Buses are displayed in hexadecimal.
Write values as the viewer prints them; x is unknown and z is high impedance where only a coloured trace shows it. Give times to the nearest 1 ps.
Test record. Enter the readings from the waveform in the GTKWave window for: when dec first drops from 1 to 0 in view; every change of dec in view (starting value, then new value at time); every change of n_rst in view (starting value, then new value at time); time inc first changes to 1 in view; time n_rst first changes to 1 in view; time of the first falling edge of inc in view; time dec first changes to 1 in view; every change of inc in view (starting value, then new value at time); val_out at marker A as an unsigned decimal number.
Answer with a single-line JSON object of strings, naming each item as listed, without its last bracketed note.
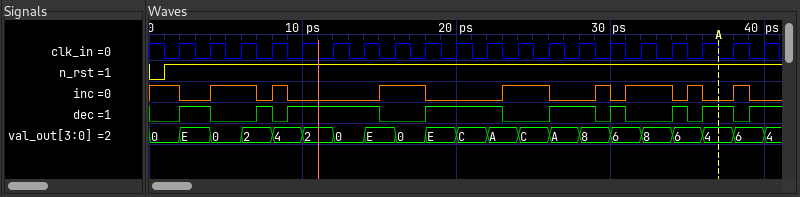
{"when dec first drops from 1 to 0 in view": "4 ps", "every change of dec in view": "0, 1 at 2 ps, 0 at 4 ps, 1 at 7 ps, 0 at 8 ps, 1 at 9 ps, 0 at 15 ps, 1 at 18 ps, 0 at 23 ps, 1 at 26 ps, 0 at 29 ps, 1 at 30 ps, 0 at 31 ps, 1 at 34 ps, 0 at 35 ps, 1 at 36 ps, 0 at 38 ps, 1 at 39 ps", "every change of n_rst in view": "0, 1 at 1 ps", "time inc first changes to 1 in view": "4 ps", "time n_rst first changes to 1 in view": "1 ps", "time of the first falling edge of inc in view": "2 ps", "time dec first changes to 1 in view": "2 ps", "every change of inc in view": "1, 0 at 2 ps, 1 at 4 ps, 0 at 7 ps, 1 at 8 ps, 0 at 9 ps, 1 at 15 ps, 0 at 18 ps, 1 at 23 ps, 0 at 26 ps, 1 at 29 ps, 0 at 30 ps, 1 at 31 ps, 0 at 34 ps, 1 at 35 ps, 0 at 36 ps, 1 at 38 ps, 0 at 39 ps", "val_out at marker A as an unsigned decimal number": "4"}
